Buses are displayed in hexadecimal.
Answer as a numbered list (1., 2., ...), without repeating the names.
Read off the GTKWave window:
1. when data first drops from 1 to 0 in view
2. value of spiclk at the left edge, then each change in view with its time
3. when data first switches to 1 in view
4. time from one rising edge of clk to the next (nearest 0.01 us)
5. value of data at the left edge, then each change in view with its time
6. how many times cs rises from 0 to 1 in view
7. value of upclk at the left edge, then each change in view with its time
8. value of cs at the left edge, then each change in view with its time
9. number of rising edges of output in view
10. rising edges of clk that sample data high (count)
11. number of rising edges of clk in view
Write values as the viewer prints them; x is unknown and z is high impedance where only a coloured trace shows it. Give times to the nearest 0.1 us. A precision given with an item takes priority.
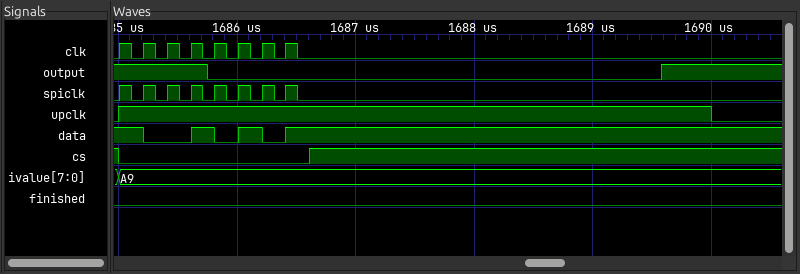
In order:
1. 1685.2 us
2. 0, 1 at 1685 us, 0 at 1685.1 us, 1 at 1685.2 us, 0 at 1685.3 us, 1 at 1685.4 us, 0 at 1685.5 us, 1 at 1685.6 us, 0 at 1685.7 us, 1 at 1685.8 us, 0 at 1685.9 us, 1 at 1686 us, 0 at 1686.1 us, 1 at 1686.2 us, 0 at 1686.3 us, 1 at 1686.4 us, 0 at 1686.5 us
3. 1685.6 us
4. 0.2 us
5. 1, 0 at 1685.2 us, 1 at 1685.6 us, 0 at 1685.8 us, 1 at 1686 us, 0 at 1686.2 us, 1 at 1686.4 us
6. 1
7. 0, 1 at 1685 us, 0 at 1690 us
8. 1, 0 at 1685 us, 1 at 1686.6 us
9. 1
10. 4
11. 8
